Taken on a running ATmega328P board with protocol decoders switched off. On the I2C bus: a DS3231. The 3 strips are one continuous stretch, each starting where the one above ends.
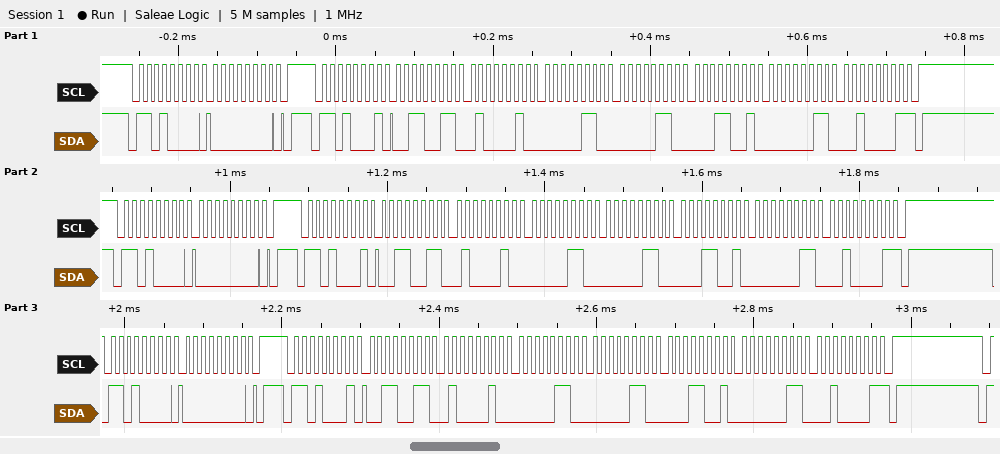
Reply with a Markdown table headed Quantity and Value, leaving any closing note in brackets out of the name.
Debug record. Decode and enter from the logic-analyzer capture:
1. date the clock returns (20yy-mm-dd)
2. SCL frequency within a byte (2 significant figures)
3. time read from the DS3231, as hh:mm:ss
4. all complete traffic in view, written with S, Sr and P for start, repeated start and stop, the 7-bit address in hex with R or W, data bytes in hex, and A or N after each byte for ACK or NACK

| Quantity | Value |
|---|---|
| date the clock returns | 2021-03-19 |
| SCL frequency within a byte | 100 kHz |
| time read from the DS3231, as hh:mm:ss | 06:42:33 |
| all complete traffic in view, written with S, Sr and P for start, repeated start and stop, the 7-bit address in hex with R or W, data bytes in hex, and A or N after each byte for ACK or NACK | S 68W A 00 A P S 68R A 33 A 42 A 06 A 06 A 19 A 03 A 21 N P S 68W A 00 A P S 68R A 33 A 42 A 06 A 06 A 19 A 03 A 21 N P S 68W A 00 A P S 68R A 33 A 42 A 06 A 06 A 19 A 03 A 21 N P |
